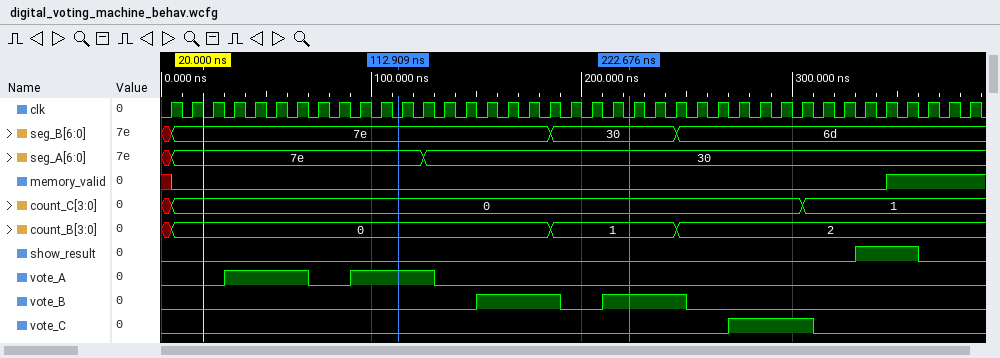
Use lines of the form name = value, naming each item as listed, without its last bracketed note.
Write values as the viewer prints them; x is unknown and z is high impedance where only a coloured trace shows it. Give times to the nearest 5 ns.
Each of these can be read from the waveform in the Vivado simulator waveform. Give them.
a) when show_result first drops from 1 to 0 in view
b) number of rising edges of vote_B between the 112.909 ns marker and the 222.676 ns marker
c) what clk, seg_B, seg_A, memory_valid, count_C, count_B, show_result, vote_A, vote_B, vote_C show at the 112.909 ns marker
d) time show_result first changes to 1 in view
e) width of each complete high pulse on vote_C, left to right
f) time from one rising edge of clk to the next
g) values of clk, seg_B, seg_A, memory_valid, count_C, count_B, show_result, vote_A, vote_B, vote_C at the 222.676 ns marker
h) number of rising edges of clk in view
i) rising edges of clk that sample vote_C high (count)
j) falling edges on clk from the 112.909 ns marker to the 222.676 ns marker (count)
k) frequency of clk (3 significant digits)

when show_result first drops from 1 to 0 in view = 360 ns
number of rising edges of vote_B between the 112.909 ns marker and the 222.676 ns marker = 2
what clk, seg_B, seg_A, memory_valid, count_C, count_B, show_result, vote_A, vote_B, vote_C show at the 112.909 ns marker = clk=0, seg_B=7e, seg_A=7e, memory_valid=0, count_C=0, count_B=0, show_result=0, vote_A=1, vote_B=0, vote_C=0
time show_result first changes to 1 in view = 330 ns
width of each complete high pulse on vote_C, left to right = 40 ns
time from one rising edge of clk to the next = 10 ns
values of clk, seg_B, seg_A, memory_valid, count_C, count_B, show_result, vote_A, vote_B, vote_C at the 222.676 ns marker = clk=0, seg_B=30, seg_A=30, memory_valid=0, count_C=0, count_B=1, show_result=0, vote_A=0, vote_B=1, vote_C=0
number of rising edges of clk in view = 39
rising edges of clk that sample vote_C high = 4
falling edges on clk from the 112.909 ns marker to the 222.676 ns marker = 11
frequency of clk = 100 MHz
